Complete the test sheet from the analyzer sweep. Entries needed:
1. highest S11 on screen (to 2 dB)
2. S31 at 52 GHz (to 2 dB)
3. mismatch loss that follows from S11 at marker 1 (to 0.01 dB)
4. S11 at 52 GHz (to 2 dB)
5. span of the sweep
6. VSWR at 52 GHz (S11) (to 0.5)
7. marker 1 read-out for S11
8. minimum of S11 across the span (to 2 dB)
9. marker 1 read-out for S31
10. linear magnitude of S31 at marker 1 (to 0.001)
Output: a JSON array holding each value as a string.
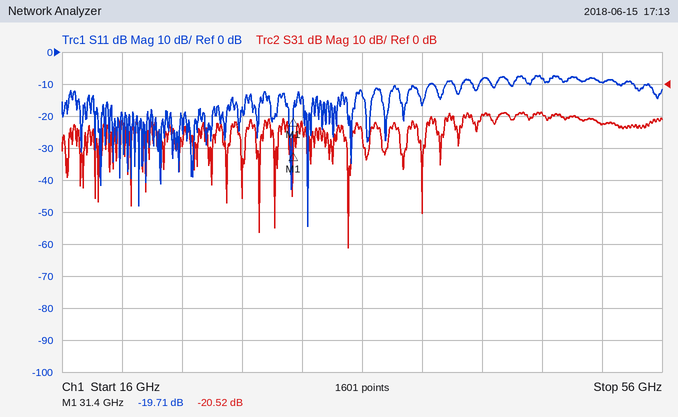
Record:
["-8 dB", "-12 dB", "0.05 dB", "-10 dB", "40 GHz", "2.0", "-19.71 dB", "-54 dB", "-20.52 dB", "0.094"]
